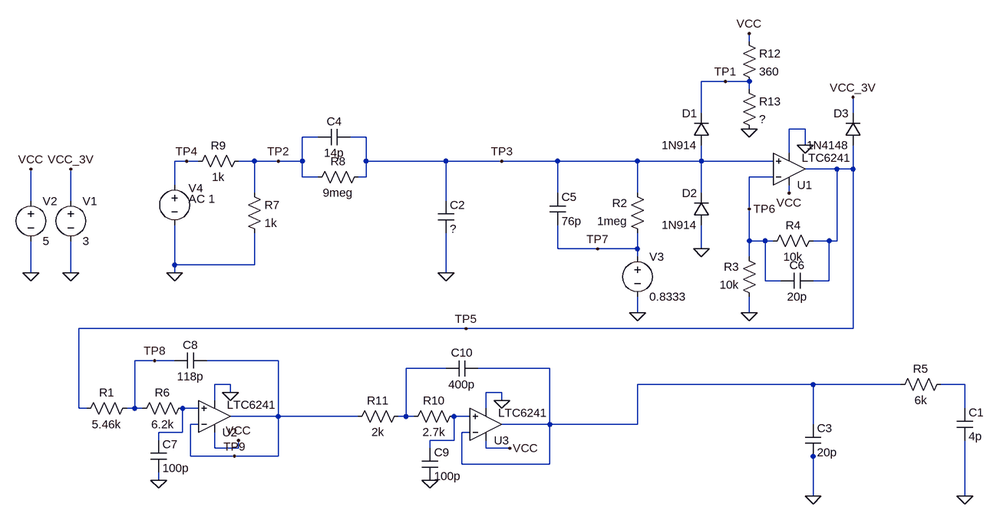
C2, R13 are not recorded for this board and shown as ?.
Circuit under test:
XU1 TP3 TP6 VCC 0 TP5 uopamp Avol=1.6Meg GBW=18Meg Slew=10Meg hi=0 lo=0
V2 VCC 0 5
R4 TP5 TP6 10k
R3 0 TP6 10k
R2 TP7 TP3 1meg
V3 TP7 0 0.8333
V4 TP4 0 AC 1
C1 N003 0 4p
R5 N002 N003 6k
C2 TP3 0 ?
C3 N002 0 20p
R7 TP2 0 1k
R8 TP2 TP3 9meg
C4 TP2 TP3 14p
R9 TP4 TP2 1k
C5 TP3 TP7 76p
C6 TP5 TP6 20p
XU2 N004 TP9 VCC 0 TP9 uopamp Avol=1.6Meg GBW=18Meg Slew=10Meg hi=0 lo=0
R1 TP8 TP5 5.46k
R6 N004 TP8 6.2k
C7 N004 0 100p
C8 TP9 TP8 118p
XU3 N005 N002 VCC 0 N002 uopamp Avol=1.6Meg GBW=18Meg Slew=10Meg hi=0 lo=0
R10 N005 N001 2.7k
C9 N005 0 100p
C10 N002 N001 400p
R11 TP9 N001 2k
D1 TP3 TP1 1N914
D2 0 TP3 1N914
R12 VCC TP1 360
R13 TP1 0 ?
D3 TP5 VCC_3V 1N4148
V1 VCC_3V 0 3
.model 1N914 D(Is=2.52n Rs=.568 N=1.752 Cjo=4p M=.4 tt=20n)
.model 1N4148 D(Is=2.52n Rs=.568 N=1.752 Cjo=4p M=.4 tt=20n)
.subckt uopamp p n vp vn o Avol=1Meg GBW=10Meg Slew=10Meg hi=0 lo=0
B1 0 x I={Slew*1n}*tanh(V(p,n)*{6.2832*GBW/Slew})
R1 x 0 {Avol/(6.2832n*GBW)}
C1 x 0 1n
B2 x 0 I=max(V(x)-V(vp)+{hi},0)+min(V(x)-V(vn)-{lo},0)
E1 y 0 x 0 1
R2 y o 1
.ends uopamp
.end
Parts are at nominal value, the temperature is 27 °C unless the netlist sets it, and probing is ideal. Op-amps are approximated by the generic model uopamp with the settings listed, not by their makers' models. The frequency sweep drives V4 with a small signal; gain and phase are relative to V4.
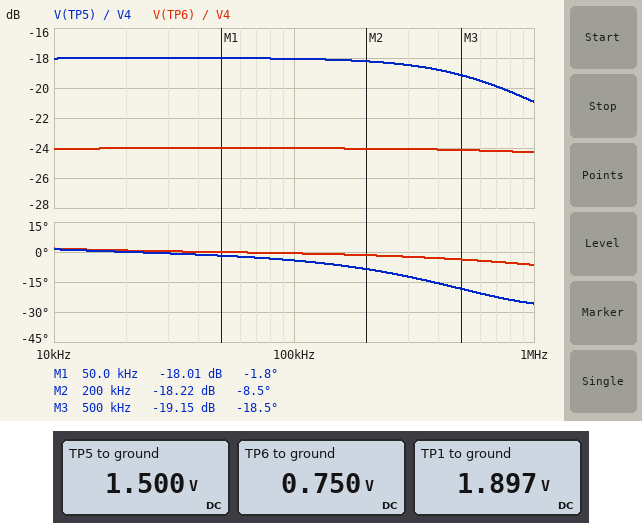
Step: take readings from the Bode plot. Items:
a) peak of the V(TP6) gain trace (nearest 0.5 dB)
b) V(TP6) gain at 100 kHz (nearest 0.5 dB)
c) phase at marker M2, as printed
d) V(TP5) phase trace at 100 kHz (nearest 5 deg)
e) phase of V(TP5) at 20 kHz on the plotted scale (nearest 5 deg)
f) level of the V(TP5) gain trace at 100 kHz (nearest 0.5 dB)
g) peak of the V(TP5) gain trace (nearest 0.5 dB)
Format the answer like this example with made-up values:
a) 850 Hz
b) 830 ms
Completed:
a) -24.0 dB
b) -24.0 dB
c) -8.5 deg
d) -5 deg
e) 0 deg
f) -18.0 dB
g) -18.0 dB
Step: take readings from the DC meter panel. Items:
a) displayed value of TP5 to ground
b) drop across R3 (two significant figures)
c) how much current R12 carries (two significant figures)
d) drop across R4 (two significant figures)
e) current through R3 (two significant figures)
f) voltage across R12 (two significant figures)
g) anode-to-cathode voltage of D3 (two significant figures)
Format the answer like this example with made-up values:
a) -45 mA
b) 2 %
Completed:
a) 1.500 V
b) 750 mV
c) 8.6 mA
d) 750 mV
e) 75 µA
f) 3.1 V
g) -1.5 V
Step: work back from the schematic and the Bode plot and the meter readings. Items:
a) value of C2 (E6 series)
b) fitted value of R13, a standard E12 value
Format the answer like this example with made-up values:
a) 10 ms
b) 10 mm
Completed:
a) 15 pF
b) 220 Ω
